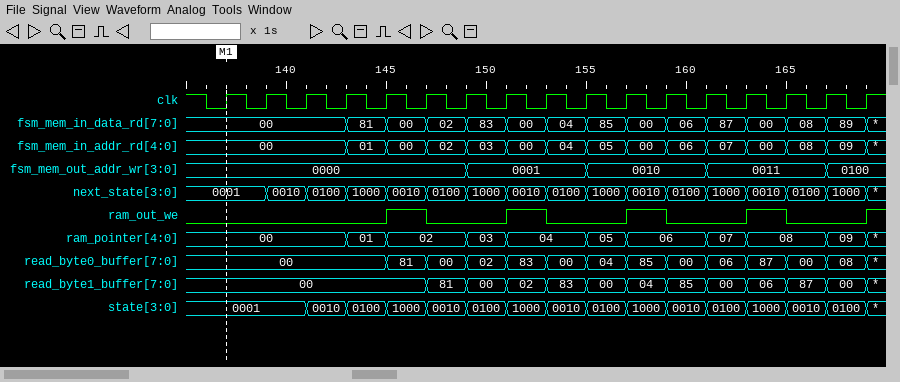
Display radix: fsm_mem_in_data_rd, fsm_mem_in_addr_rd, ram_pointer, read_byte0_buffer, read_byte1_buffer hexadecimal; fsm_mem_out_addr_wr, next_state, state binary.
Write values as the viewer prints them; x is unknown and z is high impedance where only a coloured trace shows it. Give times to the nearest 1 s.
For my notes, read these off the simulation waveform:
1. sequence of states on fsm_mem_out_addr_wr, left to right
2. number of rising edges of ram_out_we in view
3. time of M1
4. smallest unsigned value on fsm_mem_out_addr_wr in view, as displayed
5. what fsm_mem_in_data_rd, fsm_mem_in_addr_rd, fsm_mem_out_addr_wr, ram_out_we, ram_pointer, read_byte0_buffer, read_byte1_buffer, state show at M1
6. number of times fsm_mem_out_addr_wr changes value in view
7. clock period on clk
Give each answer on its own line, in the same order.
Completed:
0000, 0001, 0010, 0011, 0100
5
137 s
0000
fsm_mem_in_data_rd=00, fsm_mem_in_addr_rd=00, fsm_mem_out_addr_wr=0000, ram_out_we=0, ram_pointer=00, read_byte0_buffer=00, read_byte1_buffer=00, state=0001
4
2 s
